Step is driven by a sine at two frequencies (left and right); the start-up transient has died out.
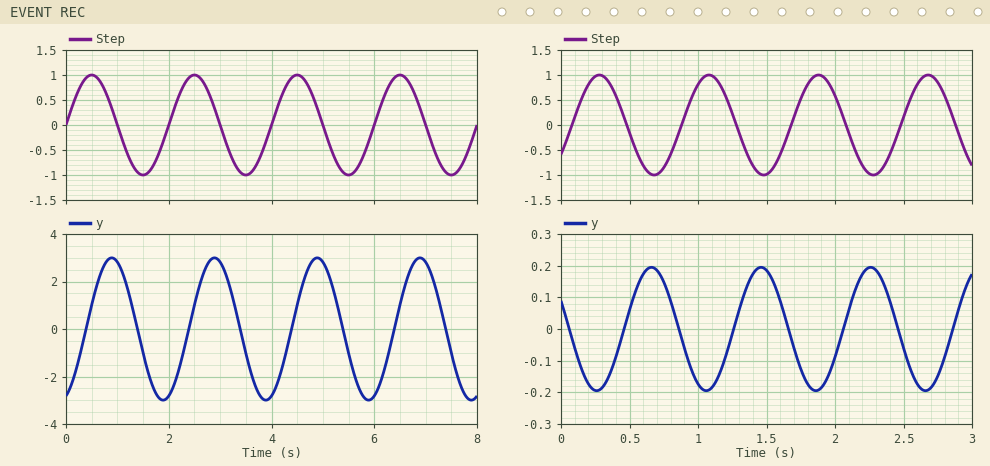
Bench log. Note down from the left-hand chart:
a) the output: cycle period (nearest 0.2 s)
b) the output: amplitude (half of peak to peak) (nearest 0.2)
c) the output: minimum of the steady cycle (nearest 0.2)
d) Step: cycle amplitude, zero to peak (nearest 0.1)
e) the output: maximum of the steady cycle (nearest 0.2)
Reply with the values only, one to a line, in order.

2.0 s
3.0
-3.0
1.0
3.0
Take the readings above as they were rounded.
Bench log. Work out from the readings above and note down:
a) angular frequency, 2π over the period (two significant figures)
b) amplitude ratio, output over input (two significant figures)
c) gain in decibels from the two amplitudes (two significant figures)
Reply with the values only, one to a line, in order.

3.1 rad/s
3.0
9.5 dB
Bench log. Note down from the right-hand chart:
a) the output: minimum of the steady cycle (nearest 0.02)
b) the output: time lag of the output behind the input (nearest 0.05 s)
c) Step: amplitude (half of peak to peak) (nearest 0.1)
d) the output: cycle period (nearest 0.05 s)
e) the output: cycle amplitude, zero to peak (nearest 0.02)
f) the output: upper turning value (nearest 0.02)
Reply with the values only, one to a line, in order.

-0.20
0.40 s
1.0
0.80 s
0.20
0.20
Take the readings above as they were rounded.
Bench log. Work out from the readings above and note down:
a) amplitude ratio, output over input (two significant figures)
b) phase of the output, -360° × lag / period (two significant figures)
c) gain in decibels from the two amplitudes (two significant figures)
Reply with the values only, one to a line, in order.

0.20
-180°
-14 dB
